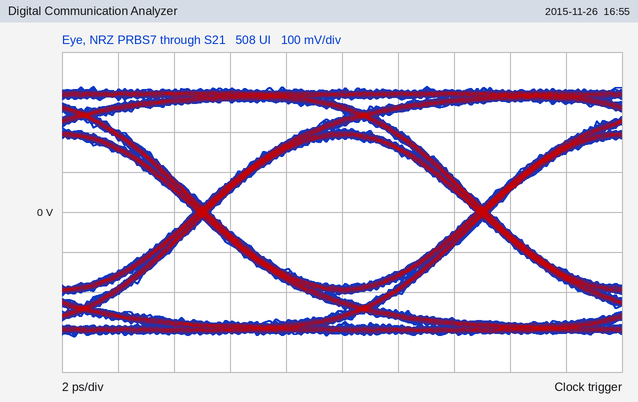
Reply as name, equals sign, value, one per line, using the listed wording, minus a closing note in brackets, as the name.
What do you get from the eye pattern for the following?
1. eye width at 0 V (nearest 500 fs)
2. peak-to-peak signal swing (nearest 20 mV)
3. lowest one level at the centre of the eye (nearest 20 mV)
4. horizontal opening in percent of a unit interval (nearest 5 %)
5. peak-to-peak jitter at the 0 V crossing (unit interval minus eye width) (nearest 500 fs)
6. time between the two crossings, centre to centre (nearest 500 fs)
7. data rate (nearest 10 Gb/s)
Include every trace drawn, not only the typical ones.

eye width at 0 V = 9.5 ps
peak-to-peak signal swing = 620 mV
lowest one level at the centre of the eye = 180 mV
horizontal opening in percent of a unit interval = 95 %
peak-to-peak jitter at the 0 V crossing (unit interval minus eye width) = 500 fs
time between the two crossings, centre to centre = 10.0 ps
data rate = 100 Gb/s
